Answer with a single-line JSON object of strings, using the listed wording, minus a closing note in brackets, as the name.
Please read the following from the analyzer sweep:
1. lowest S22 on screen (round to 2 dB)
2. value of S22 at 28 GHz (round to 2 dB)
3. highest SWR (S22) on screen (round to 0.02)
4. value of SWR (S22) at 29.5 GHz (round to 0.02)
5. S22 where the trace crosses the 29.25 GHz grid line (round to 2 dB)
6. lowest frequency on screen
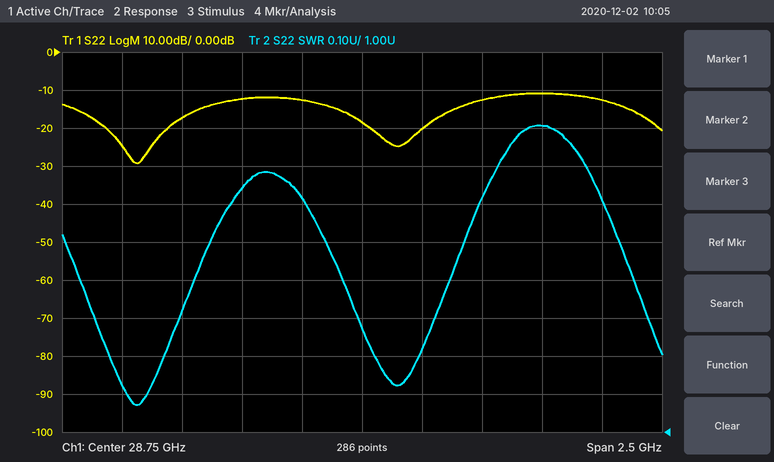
{"lowest S22 on screen": "-30 dB", "value of S22 at 28 GHz": "-18 dB", "highest SWR (S22) on screen": "1.80", "value of SWR (S22) at 29.5 GHz": "1.80", "S22 where the trace crosses the 29.25 GHz grid line": "-12 dB", "lowest frequency on screen": "27.5 GHz"}
